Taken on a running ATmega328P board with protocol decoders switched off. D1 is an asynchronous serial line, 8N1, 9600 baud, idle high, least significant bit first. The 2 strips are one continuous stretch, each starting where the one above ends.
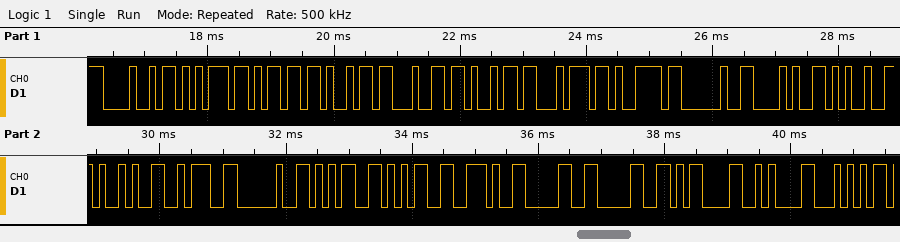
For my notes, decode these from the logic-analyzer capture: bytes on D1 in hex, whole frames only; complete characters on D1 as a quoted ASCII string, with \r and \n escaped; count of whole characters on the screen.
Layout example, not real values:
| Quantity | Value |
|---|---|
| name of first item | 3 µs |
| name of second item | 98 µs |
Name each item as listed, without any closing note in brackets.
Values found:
| Quantity | Value |
|---|---|
| bytes on D1 in hex, whole frames only | 48 75 6D 69 64 69 74 79 20 28 25 29 3A 20 35 35 2E 30 30 0D 0A 54 |
| complete characters on D1 as a quoted ASCII string, with \r and \n escaped | "Humidity (%): 55.00\r\nT" |
| count of whole characters on the screen | 22 |
